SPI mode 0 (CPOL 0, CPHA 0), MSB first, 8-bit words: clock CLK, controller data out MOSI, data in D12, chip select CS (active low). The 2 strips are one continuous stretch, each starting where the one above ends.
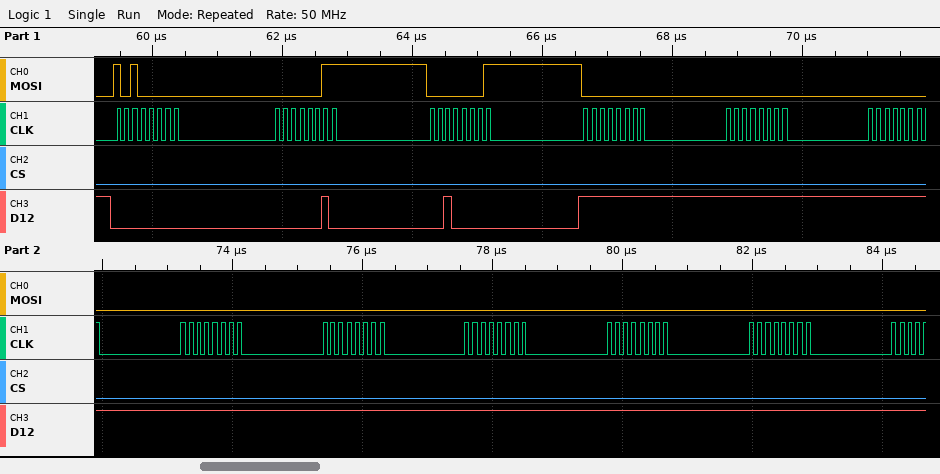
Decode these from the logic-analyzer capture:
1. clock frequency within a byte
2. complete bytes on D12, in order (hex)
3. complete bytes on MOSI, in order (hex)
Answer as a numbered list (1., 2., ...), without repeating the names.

1. 8 MHz
2. 00 02 20 FF FF FF FF FF FF FF FF
3. A0 03 01 00 00 00 00 00 00 00 00
